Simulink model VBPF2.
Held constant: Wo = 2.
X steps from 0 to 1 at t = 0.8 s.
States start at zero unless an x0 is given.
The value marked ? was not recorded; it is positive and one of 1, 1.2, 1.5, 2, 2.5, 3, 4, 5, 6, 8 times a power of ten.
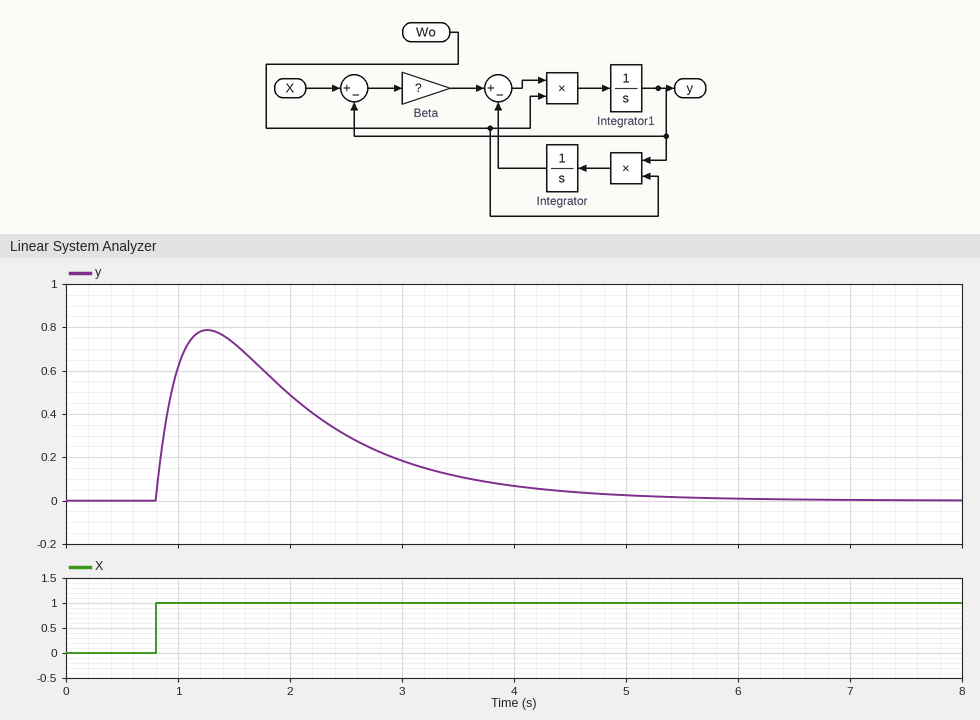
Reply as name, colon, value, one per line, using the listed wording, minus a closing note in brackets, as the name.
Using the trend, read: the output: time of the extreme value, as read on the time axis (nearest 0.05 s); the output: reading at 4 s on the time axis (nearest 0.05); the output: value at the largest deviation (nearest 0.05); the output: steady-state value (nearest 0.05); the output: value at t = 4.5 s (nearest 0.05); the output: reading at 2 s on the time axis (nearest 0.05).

the output: time of the extreme value, as read on the time axis: 1.25 s
the output: reading at 4 s on the time axis: 0.05
the output: value at the largest deviation: 0.80
the output: steady-state value: 0.00
the output: value at t = 4.5 s: 0.05
the output: reading at 2 s on the time axis: 0.50
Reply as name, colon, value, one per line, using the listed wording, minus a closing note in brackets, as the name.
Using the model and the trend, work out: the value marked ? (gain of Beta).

the value marked ?: 2.5
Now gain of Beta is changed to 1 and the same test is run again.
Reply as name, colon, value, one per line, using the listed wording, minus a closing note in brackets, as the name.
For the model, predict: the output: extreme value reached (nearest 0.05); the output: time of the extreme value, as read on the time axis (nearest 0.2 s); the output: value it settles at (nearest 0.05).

the output: extreme value reached: 0.55
the output: time of the extreme value, as read on the time axis: 1.4 s
the output: value it settles at: 0.00
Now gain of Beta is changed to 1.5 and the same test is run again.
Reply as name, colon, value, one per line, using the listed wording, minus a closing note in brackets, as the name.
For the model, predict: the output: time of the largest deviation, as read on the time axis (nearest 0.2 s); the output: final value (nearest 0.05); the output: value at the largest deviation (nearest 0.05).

the output: time of the largest deviation, as read on the time axis: 1.4 s
the output: final value: 0.00
the output: value at the largest deviation: 0.65
